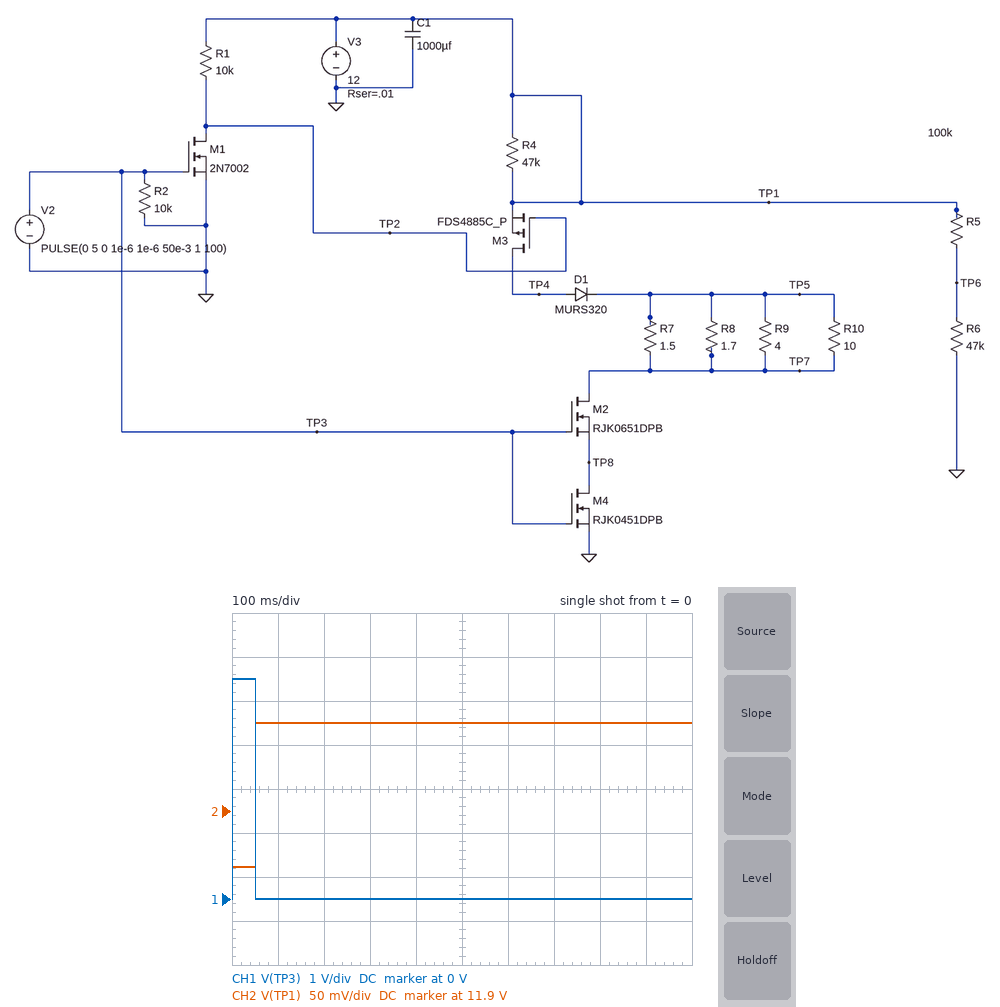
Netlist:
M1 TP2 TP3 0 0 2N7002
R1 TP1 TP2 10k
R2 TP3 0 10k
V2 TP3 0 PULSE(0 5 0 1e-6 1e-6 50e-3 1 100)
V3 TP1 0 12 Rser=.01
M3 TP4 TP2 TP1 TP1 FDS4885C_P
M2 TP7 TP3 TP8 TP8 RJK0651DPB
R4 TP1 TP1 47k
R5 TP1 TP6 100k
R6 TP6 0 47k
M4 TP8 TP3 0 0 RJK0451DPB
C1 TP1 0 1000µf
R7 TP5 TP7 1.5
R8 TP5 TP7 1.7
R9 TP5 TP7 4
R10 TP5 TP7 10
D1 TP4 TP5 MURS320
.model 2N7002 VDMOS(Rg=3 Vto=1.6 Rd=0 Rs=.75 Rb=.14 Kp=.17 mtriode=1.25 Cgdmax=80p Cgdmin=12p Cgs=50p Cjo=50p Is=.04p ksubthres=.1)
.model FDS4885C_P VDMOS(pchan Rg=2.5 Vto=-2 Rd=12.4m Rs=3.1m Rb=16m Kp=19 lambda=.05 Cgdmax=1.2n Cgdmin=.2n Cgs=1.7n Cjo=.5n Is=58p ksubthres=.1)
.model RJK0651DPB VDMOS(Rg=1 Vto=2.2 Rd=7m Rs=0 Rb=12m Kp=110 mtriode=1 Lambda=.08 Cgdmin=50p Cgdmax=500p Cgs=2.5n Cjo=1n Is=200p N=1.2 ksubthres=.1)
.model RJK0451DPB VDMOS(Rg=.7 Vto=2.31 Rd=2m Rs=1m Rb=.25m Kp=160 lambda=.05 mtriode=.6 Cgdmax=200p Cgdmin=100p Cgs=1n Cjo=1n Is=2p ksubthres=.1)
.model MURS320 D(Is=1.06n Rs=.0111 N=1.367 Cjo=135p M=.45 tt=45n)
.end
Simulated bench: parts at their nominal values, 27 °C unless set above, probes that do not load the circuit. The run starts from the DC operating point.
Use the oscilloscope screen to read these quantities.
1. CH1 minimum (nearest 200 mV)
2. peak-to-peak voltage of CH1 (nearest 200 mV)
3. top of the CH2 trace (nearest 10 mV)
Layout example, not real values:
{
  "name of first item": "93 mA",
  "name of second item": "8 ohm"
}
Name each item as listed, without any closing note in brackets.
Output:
{
  "CH1 minimum": "0 V",
  "peak-to-peak voltage of CH1": "5.0 V",
  "top of the CH2 trace": "12.00 V"
}
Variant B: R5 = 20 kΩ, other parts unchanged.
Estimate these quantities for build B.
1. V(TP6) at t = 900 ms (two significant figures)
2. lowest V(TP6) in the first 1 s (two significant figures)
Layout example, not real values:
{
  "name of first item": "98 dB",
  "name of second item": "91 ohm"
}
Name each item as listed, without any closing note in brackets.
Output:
{
  "V(TP6) at t = 900 ms": "8.4 V",
  "lowest V(TP6) in the first 1 s": "8.3 V"
}
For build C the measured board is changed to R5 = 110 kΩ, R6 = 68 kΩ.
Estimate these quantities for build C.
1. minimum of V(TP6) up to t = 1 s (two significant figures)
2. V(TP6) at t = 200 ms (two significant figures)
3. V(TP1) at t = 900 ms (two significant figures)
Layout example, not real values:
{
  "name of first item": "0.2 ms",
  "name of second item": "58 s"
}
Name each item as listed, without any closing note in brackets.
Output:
{
  "minimum of V(TP6) up to t = 1 s": "4.5 V",
  "V(TP6) at t = 200 ms": "4.6 V",
  "V(TP1) at t = 900 ms": "12 V"
}
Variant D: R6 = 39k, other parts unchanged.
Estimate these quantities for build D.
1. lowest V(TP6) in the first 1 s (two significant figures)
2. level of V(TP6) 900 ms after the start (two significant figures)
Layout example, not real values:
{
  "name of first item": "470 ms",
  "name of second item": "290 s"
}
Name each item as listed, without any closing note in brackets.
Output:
{
  "lowest V(TP6) in the first 1 s": "3.3 V",
  "level of V(TP6) 900 ms after the start": "3.4 V"
}
